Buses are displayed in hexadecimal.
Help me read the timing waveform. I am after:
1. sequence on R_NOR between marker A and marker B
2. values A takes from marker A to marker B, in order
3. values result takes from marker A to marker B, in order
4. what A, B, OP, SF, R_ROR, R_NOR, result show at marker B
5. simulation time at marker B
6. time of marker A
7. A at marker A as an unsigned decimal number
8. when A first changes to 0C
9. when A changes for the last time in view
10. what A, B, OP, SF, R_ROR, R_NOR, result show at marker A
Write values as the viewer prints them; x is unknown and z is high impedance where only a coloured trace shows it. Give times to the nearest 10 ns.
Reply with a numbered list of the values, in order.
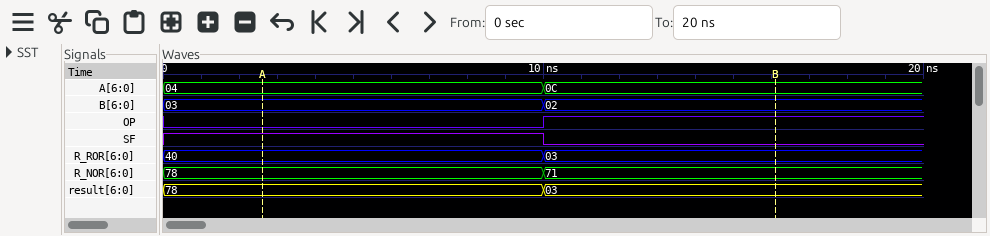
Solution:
1. 78, 71
2. 04, 0C
3. 78, 03
4. A=0C, B=02, OP=1, SF=0, R_ROR=03, R_NOR=71, result=03
5. 20 ns
6. 0 ns
7. 4
8. 10 ns
9. 10 ns
10. A=04, B=03, OP=0, SF=1, R_ROR=40, R_NOR=78, result=78
